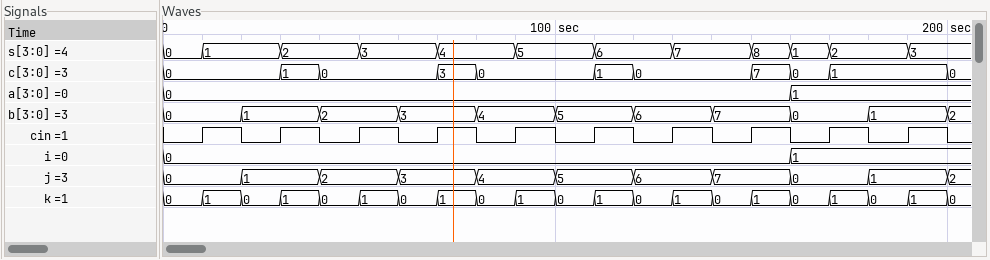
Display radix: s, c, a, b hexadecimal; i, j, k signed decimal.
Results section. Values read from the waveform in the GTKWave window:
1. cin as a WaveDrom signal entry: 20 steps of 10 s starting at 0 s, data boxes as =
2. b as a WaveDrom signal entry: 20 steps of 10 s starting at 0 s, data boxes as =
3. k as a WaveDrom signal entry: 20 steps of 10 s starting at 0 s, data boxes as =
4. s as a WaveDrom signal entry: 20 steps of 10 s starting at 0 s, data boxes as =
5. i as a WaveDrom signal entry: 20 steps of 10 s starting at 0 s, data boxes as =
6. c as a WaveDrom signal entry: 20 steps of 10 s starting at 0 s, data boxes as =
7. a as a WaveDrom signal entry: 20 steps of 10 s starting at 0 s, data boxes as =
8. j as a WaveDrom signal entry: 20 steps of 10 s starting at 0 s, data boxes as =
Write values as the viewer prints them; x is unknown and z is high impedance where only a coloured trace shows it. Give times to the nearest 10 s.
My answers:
{name: 'cin', wave: '01010101010101010101'}
{name: 'b', wave: '=.=.=.=.=.=.=.=.=.=.', data: '0 1 2 3 4 5 6 7 0 1'}
{name: 'k', wave: '====================', data: '0 1 0 1 0 1 0 1 0 1 0 1 0 1 0 1 0 1 0 1'}
{name: 's', wave: '==.=.=.=.=.=.=.===.=', data: '0 1 2 3 4 5 6 7 8 1 2 3'}
{name: 'i', wave: '=...............=...', data: '0 1'}
{name: 'c', wave: '=..==..==..==..===..', data: '0 1 0 3 0 1 0 7 0 1'}
{name: 'a', wave: '=...............=...', data: '0 1'}
{name: 'j', wave: '=.=.=.=.=.=.=.=.=.=.', data: '0 1 2 3 4 5 6 7 0 1'}
